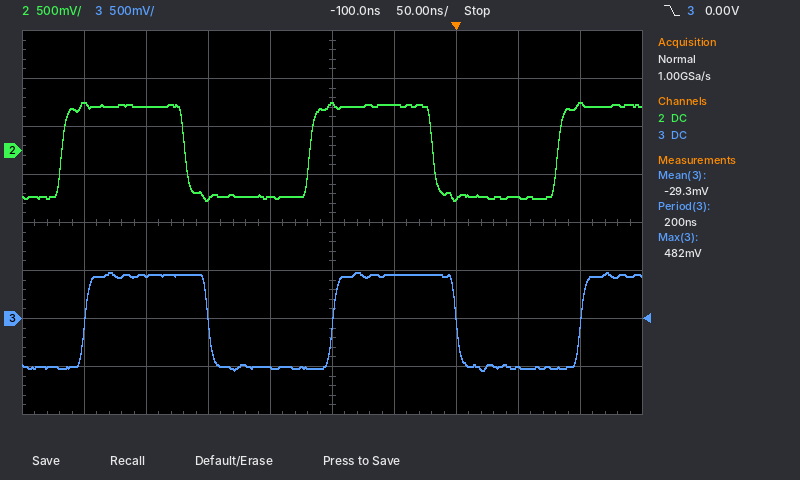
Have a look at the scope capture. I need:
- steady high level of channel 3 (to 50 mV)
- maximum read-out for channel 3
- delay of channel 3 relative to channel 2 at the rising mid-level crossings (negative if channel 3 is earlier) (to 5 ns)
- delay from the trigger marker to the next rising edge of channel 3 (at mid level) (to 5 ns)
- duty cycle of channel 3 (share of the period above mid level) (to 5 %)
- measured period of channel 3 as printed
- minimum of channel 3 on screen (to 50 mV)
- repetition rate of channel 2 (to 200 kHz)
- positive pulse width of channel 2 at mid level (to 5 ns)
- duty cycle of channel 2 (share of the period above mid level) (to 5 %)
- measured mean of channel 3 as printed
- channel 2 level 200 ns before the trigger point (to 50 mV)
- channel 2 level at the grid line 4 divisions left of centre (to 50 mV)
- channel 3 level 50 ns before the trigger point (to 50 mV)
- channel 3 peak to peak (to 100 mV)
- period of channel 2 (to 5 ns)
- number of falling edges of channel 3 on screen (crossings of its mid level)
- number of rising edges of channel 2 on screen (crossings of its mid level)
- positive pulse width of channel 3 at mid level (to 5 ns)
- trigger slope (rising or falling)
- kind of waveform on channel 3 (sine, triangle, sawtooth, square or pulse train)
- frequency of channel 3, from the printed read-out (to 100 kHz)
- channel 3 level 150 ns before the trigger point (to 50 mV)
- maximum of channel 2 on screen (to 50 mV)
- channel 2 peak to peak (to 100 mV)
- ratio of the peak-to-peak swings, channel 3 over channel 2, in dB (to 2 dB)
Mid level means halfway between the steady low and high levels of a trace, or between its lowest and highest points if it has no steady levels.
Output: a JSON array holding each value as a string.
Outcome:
["450 mV", "482 mV", "+20 ns", "100 ns", "50 %", "200 ns", "-550 mV", "5.0 MHz", "100 ns", "50 %", "-29.3 mV", "-500 mV", "500 mV", "450 mV", "1.00 V", "200 ns", "2", "3", "100 ns", "falling", "square", "5.0 MHz", "-500 mV", "500 mV", "1.00 V", "0 dB"]
